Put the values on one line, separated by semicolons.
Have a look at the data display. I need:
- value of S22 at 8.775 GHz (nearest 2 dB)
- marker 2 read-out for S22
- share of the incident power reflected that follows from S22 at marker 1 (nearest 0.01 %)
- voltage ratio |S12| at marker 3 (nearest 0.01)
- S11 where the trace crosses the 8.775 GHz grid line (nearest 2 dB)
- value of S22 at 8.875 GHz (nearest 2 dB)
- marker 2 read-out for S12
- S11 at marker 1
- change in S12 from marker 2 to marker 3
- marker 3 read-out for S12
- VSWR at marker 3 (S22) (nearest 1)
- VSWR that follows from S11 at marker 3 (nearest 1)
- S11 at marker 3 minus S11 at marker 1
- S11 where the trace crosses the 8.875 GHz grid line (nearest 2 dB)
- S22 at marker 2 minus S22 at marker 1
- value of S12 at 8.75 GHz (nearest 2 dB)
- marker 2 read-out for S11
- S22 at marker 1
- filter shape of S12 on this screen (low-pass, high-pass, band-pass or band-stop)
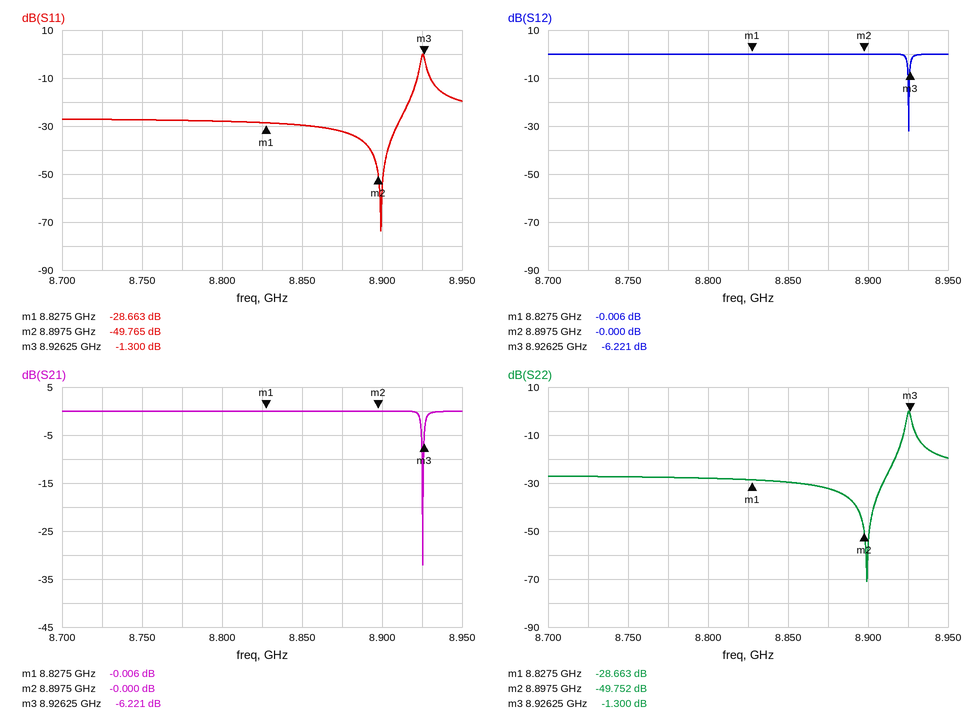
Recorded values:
-28 dB; -49.752 dB; 0.14 %; 0.49; -28 dB; -32 dB; -0.000 dB; -28.663 dB; -6.221 dB; -6.221 dB; 13; 13; 27.363 dB; -32 dB; -21.089 dB; 0 dB; -49.765 dB; -28.663 dB; band-stop
